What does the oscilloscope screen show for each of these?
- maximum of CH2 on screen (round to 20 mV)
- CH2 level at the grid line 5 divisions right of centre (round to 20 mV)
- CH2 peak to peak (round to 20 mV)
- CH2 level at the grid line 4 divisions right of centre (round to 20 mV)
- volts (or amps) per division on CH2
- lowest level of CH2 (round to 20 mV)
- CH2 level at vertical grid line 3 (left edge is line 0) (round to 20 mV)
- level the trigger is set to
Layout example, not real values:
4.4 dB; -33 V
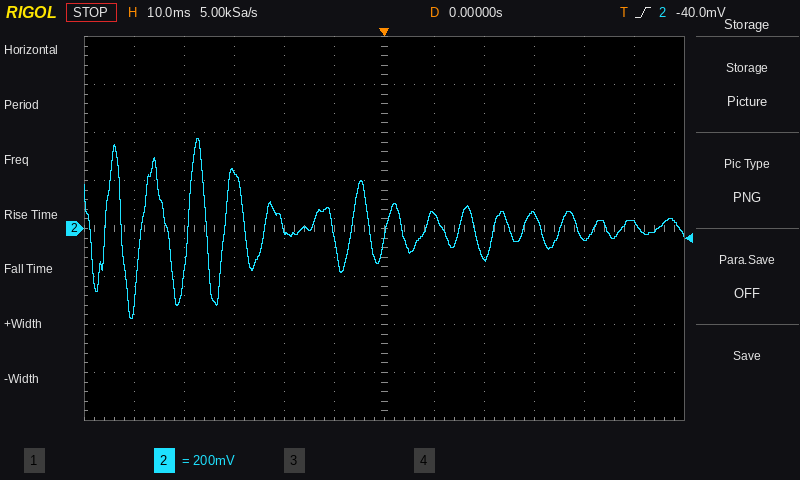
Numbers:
380 mV; 20 mV; 760 mV; -40 mV; 200 mV; -380 mV; 240 mV; -40.0 mV
